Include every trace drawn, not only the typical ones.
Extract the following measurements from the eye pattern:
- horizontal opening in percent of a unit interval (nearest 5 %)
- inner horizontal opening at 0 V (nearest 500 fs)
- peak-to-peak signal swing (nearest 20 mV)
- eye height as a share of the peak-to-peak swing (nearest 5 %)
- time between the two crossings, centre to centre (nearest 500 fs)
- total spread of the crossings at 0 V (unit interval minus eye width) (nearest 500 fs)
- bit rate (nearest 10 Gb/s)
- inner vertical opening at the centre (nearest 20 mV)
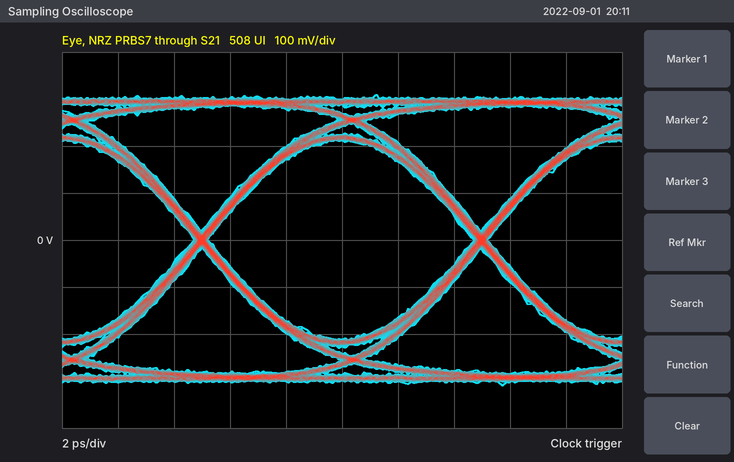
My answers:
95 %
9.5 ps
620 mV
70 %
10.0 ps
500 fs
100 Gb/s
420 mV
